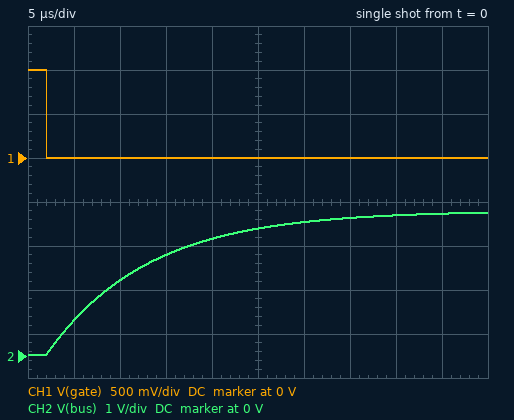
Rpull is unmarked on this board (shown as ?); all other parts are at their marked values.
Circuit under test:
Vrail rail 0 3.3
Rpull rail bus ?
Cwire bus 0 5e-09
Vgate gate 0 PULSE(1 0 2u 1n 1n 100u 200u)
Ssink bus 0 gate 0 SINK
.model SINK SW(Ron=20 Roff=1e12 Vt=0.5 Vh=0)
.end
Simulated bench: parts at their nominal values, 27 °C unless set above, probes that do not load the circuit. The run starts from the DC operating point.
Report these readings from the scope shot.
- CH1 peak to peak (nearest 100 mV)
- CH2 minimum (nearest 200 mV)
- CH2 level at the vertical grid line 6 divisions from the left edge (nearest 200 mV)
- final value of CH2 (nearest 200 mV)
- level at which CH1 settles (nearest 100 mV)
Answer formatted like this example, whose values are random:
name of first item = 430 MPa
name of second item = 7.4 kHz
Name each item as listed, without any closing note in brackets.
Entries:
CH1 peak to peak = 1.0 V
CH2 minimum = 0 V
CH2 level at the vertical grid line 6 divisions from the left edge = 3.0 V
final value of CH2 = 3.2 V
level at which CH1 settles = 0 V
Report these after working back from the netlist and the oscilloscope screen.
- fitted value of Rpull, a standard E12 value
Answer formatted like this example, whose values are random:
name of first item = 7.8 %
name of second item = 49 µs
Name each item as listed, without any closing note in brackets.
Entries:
fitted value of Rpull, a standard E12 value = 2.2 kΩ
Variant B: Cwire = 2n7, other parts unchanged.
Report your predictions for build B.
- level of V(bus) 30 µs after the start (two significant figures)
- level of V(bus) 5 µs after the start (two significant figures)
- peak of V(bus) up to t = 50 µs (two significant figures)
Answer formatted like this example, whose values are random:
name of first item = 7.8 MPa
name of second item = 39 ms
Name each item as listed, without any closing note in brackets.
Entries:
level of V(bus) 30 µs after the start = 3.3 V
level of V(bus) 5 µs after the start = 1.3 V
peak of V(bus) up to t = 50 µs = 3.3 V
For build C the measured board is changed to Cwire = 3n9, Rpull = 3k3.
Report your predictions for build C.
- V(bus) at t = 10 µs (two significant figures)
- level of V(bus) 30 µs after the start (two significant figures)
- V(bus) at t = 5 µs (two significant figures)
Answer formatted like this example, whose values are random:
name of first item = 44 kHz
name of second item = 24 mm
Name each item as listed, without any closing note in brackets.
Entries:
V(bus) at t = 10 µs = 1.5 V
level of V(bus) 30 µs after the start = 2.9 V
V(bus) at t = 5 µs = 700 mV
